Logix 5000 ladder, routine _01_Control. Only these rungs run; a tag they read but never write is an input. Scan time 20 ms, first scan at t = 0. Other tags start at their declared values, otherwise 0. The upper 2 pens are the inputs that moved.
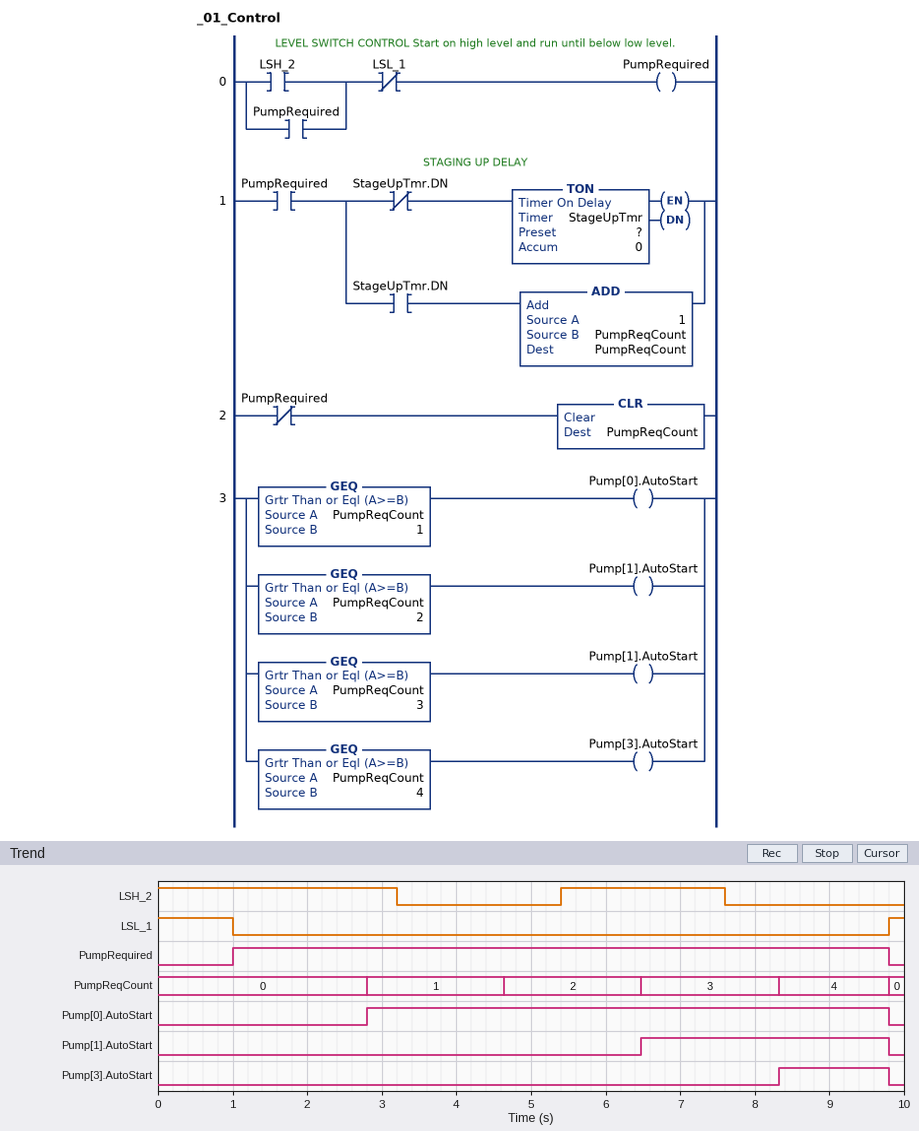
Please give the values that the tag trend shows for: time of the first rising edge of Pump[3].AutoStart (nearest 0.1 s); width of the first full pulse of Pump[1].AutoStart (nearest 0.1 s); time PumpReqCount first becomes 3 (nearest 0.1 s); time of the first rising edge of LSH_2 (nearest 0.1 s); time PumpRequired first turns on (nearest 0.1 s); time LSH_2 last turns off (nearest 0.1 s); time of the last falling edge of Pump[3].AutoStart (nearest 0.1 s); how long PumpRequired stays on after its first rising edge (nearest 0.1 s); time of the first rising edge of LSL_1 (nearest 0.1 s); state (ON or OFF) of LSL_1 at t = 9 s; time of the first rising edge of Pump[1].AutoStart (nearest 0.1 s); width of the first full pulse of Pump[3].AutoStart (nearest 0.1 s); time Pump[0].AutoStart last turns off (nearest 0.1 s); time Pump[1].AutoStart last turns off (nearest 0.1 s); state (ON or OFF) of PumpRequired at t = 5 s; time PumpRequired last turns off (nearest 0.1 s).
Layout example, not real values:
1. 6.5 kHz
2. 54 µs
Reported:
1. 8.3 s
2. 3.3 s
3. 6.5 s
4. 5.4 s
5. 1.0 s
6. 7.6 s
7. 9.8 s
8. 8.8 s
9. 9.8 s
10. OFF
11. 6.5 s
12. 1.5 s
13. 9.8 s
14. 9.8 s
15. ON
16. 9.8 s
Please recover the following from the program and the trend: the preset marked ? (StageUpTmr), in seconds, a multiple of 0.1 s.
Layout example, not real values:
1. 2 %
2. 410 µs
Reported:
1. 1.8 s
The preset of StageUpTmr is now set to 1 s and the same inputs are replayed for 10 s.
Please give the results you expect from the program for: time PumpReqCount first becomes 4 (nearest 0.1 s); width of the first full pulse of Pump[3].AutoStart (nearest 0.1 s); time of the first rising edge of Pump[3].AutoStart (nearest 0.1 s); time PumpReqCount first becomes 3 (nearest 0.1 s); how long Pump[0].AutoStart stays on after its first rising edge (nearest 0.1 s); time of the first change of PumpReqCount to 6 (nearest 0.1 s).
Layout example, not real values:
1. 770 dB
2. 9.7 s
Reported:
1. 5.1 s
2. 4.7 s
3. 5.1 s
4. 4.1 s
5. 7.8 s
6. 7.2 s
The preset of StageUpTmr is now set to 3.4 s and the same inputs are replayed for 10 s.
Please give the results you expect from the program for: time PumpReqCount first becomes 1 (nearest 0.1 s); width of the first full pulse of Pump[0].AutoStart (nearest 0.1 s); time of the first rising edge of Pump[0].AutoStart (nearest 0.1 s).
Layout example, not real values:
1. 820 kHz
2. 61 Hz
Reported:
1. 4.4 s
2. 5.4 s
3. 4.4 s
